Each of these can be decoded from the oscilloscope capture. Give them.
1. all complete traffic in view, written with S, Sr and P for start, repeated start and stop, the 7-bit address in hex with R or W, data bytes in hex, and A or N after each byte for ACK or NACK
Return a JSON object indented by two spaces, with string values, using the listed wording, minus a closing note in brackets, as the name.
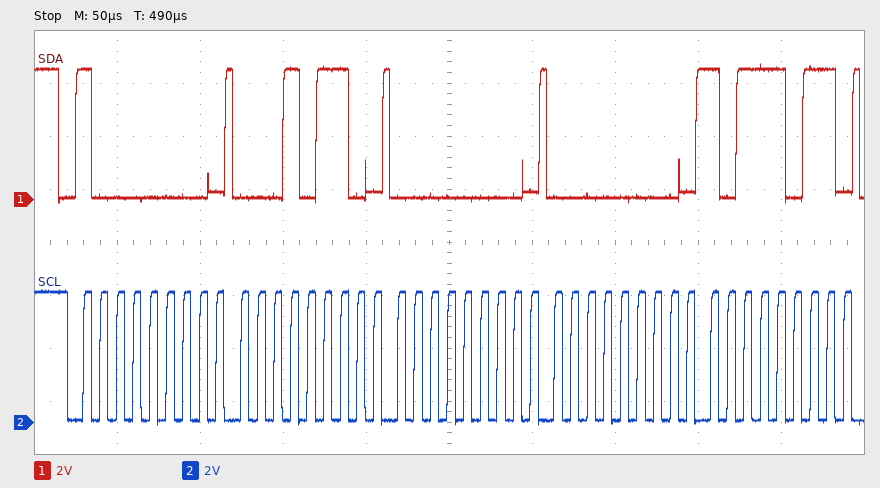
{
  "all complete traffic in view, written with S, Sr and P for start, repeated start and stop, the 7-bit address in hex with R or W, data bytes in hex, and A or N after each byte for ACK or NACK": "S 40W A 16 A 00 A 00 A BB A"
}
